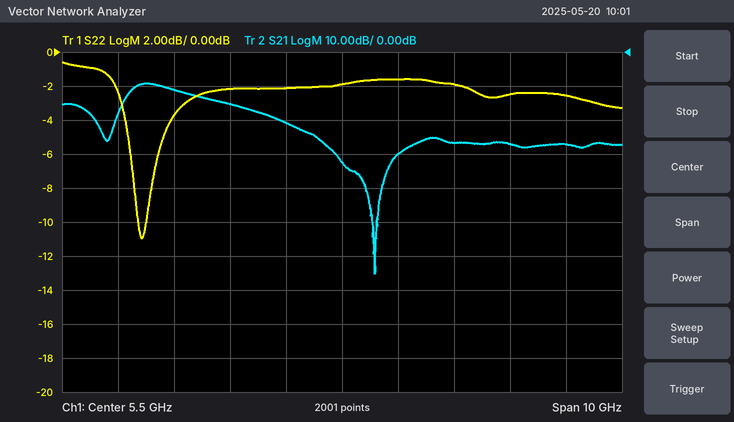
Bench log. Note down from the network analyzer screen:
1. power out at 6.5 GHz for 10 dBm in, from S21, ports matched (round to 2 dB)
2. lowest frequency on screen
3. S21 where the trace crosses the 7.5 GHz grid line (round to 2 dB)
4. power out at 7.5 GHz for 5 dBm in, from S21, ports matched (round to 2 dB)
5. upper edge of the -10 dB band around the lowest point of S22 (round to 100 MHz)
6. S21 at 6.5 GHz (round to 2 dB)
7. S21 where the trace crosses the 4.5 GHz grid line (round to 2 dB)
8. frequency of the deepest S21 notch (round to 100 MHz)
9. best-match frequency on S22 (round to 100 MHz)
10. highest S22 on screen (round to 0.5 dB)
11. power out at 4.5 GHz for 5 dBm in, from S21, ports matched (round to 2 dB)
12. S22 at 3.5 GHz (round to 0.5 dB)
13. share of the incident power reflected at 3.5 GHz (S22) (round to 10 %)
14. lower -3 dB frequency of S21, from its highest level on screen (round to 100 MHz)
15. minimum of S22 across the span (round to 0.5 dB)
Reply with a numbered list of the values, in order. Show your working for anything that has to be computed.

1. 10 dBm + (-30 dB) = -20 dBm
2. 500 MHz
3. -26 dB
4. 5 dBm + (-26 dB) = -22 dBm
5. 2.0 GHz
6. -30 dB
7. -20 dB
8. 6.1 GHz
9. 1.9 GHz
10. -0.5 dB
11. 5 dBm + (-20 dB) = -16 dBm
12. -2.0 dB
13. 10^(-2/10) ≈ 63.1 %, so 60 % to the nearest 10 %
14. 1.7 GHz
15. -11.0 dB
